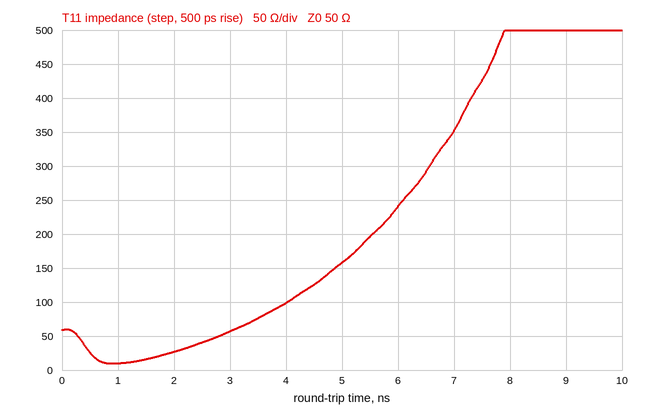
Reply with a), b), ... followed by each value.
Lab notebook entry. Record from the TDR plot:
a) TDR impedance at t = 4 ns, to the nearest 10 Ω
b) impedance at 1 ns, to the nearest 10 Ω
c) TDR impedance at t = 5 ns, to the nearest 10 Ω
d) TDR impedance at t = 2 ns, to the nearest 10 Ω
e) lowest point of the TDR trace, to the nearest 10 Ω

a) 100 Ω
b) 10 Ω
c) 160 Ω
d) 30 Ω
e) 10 Ω
